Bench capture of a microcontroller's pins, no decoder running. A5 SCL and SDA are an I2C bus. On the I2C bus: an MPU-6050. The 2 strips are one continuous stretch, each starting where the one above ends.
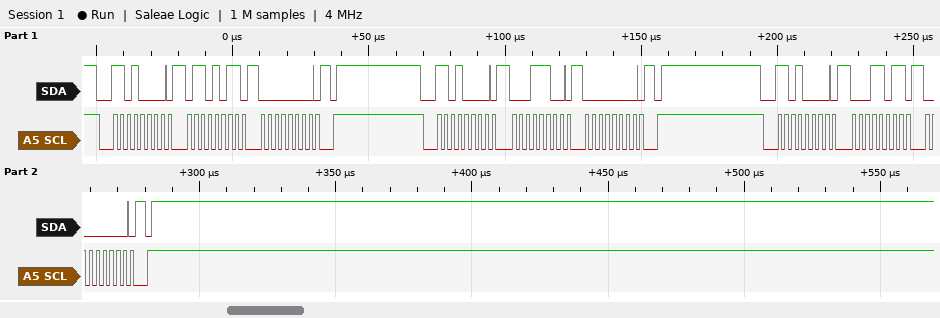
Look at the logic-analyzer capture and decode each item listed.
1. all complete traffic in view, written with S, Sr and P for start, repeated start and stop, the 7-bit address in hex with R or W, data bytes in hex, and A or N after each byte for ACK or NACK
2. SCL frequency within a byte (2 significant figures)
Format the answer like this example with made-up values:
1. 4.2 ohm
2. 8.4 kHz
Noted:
1. S 68W A 6B A 00 A P S 68W A 1C A 00 A P S 68W A 1B A 00 A P
2. 400 kHz
